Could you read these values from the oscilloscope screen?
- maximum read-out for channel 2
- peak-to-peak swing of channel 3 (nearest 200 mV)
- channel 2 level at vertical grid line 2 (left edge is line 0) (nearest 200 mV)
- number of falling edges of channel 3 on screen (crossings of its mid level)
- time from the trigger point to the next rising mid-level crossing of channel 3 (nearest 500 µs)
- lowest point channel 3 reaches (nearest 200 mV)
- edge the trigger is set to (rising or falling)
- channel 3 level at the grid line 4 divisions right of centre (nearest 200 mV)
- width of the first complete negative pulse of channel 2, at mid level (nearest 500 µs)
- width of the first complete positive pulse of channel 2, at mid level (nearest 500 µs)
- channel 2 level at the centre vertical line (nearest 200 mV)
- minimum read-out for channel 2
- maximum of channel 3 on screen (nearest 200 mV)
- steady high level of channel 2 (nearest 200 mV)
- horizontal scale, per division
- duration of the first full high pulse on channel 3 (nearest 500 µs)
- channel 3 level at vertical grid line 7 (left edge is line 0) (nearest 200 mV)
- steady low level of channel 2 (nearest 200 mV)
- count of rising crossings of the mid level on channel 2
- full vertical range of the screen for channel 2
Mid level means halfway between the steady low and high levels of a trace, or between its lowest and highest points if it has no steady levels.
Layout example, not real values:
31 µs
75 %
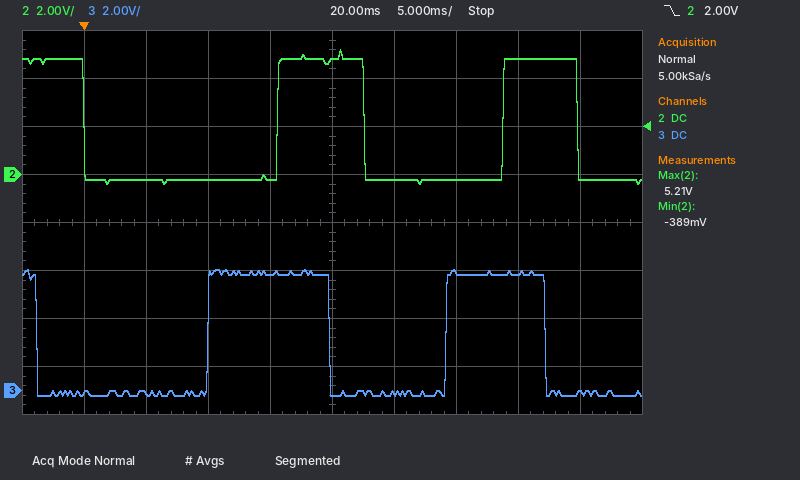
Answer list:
5.21 V
5.2 V
-200 mV
3
10.0 ms
-200 mV
falling
0.0 V
15.5 ms
7.0 ms
4.8 V
-389 mV
5.0 V
4.8 V
5 ms
10.0 ms
5.0 V
-200 mV
2
16 V
